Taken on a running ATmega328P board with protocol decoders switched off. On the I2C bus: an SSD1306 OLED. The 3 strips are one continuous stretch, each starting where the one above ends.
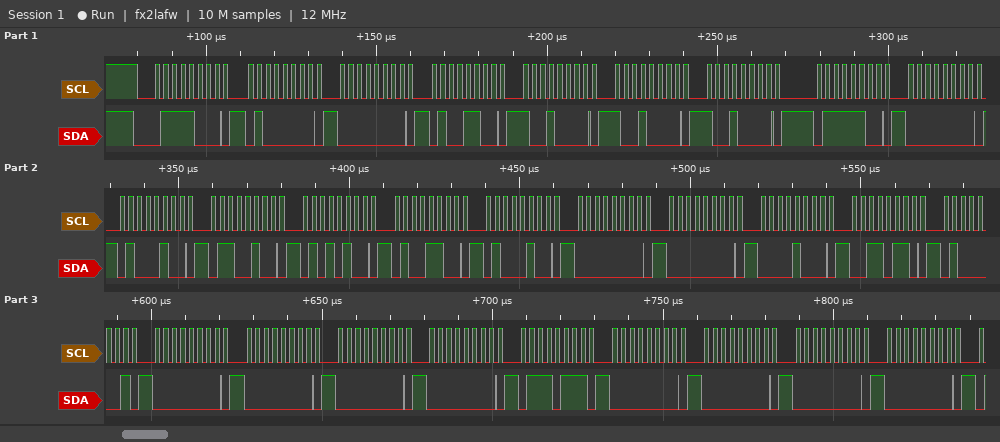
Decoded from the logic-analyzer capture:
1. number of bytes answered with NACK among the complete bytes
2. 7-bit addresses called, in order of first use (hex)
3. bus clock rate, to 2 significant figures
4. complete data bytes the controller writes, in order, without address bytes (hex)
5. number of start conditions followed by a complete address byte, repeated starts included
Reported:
0
0x3C
400 kHz
40 00 4C 90 90 90 7C 00 44 64 54 4C 44 00 00 08 36 41 00 00 00 00 77 00 00 00 00
1
